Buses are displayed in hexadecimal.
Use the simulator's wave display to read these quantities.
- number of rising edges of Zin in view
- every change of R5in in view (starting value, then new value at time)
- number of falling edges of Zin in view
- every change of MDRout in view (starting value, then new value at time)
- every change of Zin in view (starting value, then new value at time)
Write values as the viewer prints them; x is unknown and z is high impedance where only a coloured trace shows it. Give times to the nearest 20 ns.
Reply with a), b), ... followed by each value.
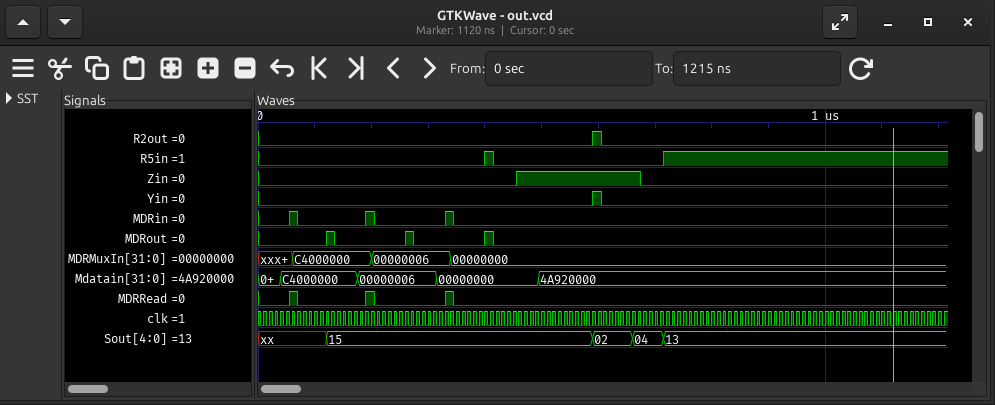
a) 1
b) 0, 1 at 400 ns, 0 at 420 ns, 1 at 720 ns
c) 1
d) 0, 1 at 120 ns, 0 at 140 ns, 1 at 260 ns, 0 at 280 ns, 1 at 400 ns, 0 at 420 ns
e) 0, 1 at 460 ns, 0 at 680 ns
